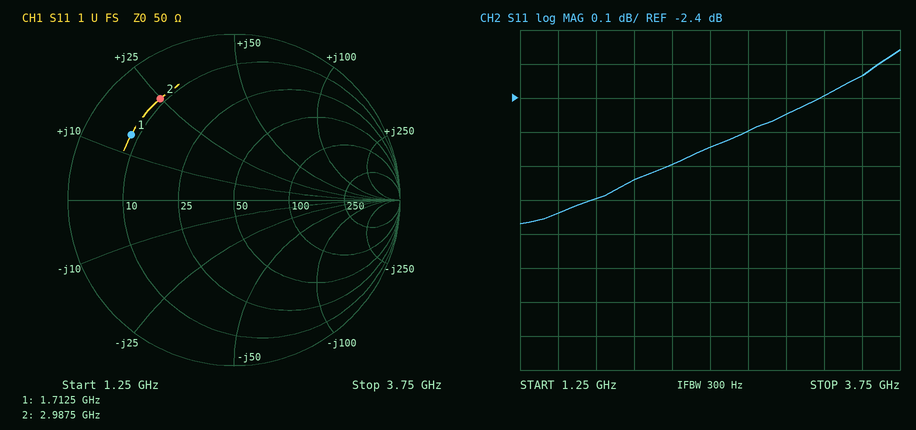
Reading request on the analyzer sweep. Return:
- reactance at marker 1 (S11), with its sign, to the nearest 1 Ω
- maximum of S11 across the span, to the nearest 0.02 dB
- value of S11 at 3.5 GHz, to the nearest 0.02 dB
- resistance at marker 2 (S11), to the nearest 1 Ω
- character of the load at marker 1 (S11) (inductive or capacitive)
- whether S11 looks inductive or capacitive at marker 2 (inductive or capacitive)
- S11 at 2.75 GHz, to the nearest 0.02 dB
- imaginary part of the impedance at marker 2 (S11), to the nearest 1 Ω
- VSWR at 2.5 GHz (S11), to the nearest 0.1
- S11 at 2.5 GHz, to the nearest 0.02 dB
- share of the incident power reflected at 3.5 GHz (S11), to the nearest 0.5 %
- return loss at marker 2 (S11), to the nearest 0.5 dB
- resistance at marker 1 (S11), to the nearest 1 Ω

+14 Ω
-2.26 dB
-2.34 dB
9 Ω
inductive
inductive
-2.50 dB
+25 Ω
6.9
-2.54 dB
58.5 %
2.5 dB
8 Ω
